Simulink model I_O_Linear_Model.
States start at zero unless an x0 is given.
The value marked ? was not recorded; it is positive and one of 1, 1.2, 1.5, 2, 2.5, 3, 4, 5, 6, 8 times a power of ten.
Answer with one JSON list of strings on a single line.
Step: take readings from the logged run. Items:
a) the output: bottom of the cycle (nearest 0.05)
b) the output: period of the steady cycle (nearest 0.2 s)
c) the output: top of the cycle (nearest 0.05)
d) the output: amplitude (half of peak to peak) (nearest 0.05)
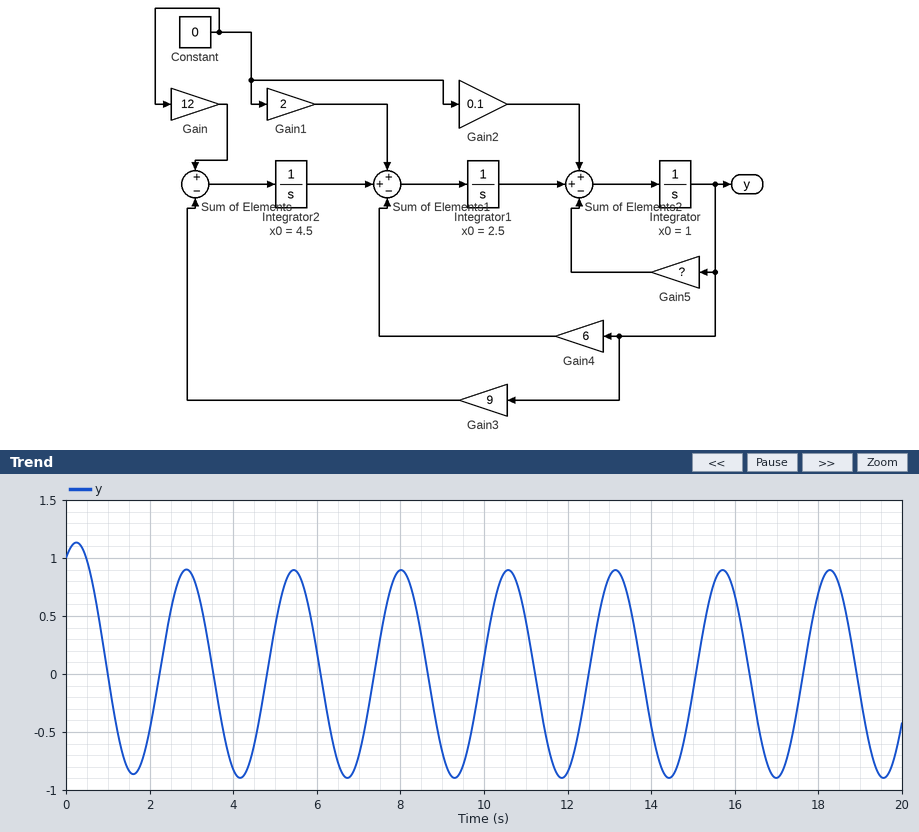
["-0.90", "2.6 s", "0.90", "0.90"]
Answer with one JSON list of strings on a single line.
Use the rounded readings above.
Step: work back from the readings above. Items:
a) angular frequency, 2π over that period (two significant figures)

["2.4 rad/s"]
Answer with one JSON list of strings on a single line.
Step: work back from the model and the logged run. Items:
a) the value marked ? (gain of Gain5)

["1.5"]
